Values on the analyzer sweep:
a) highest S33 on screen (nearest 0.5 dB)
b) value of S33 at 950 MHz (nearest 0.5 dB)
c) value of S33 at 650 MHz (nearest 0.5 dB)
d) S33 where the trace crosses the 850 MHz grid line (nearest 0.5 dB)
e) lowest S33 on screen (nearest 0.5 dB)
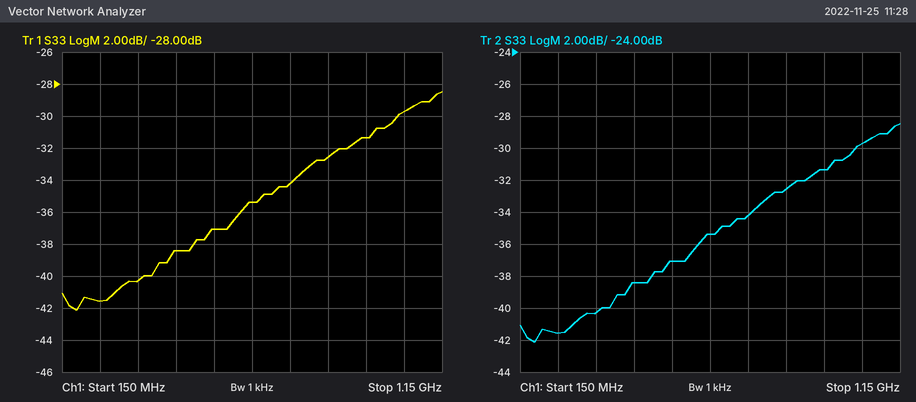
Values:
-28.5 dB
-31.5 dB
-35.5 dB
-32.5 dB
-42.0 dB
